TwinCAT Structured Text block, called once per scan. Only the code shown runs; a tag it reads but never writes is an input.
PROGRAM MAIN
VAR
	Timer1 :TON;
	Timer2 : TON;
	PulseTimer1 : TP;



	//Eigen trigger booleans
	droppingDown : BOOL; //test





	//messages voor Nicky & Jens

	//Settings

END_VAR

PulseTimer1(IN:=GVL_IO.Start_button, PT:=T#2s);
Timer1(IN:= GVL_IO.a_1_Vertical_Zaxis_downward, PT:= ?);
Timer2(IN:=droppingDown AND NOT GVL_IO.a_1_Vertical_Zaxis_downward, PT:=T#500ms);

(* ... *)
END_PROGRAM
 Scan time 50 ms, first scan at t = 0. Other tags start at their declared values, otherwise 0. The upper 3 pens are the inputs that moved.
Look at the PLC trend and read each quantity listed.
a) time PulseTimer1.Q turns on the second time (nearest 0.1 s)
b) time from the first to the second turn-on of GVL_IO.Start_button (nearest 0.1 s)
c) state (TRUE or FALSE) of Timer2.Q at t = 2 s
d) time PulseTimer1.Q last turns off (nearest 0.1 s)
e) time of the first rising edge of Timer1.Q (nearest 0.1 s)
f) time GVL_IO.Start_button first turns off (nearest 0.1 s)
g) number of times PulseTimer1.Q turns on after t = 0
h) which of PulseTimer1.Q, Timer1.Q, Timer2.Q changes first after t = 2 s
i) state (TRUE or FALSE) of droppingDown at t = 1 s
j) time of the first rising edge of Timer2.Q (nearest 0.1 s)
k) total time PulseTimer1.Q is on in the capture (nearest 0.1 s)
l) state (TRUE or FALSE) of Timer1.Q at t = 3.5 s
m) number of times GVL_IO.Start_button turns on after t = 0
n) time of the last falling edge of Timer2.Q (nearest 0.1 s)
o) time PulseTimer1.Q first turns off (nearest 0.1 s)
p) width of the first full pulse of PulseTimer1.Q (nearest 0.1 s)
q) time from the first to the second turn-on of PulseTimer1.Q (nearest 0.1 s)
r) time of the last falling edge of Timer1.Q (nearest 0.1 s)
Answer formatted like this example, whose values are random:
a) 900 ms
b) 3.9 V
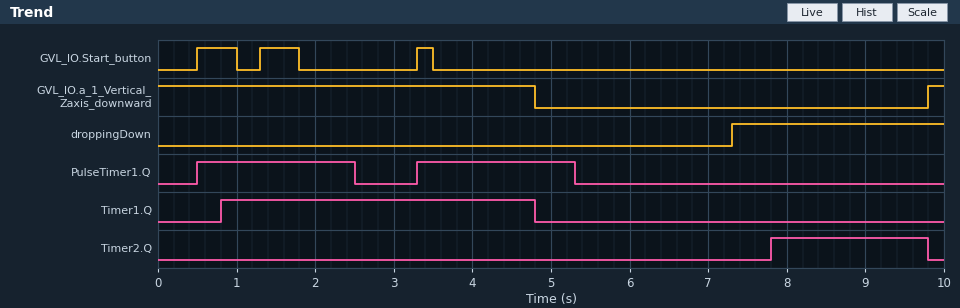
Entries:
a) 3.3 s
b) 0.8 s
c) FALSE
d) 5.3 s
e) 0.8 s
f) 1.0 s
g) 2
h) PulseTimer1.Q
i) FALSE
j) 7.8 s
k) 4.0 s
l) TRUE
m) 3
n) 9.8 s
o) 2.5 s
p) 2.0 s
q) 2.8 s
r) 4.8 s
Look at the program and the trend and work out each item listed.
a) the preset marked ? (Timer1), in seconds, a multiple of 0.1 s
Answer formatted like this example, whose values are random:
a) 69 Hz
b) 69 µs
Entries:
a) 0.8 s
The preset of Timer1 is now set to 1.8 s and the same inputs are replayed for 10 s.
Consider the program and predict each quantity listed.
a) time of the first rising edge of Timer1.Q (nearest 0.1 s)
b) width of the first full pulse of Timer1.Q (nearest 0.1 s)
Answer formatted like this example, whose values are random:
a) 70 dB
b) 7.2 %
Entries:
a) 1.8 s
b) 3.0 s
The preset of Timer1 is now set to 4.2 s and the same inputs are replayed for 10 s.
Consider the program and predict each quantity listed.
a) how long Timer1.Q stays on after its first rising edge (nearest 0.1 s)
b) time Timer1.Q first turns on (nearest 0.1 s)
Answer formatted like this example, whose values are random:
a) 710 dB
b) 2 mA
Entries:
a) 0.6 s
b) 4.2 s
